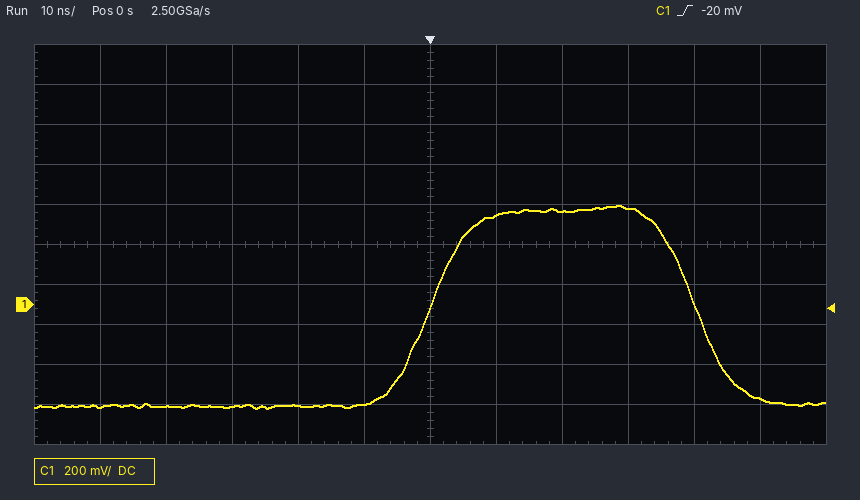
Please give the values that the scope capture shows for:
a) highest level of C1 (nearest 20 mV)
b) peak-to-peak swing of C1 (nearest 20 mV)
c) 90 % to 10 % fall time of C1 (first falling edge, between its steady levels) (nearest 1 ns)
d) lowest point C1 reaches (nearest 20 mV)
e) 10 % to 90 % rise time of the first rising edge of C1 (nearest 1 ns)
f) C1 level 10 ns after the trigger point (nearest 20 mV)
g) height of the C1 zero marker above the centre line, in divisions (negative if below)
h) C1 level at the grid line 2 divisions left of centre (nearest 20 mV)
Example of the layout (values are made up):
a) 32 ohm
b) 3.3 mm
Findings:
a) 500 mV
b) 1.02 V
c) 12 ns
d) -520 mV
e) 12 ns
f) 440 mV
g) -1.5 div
h) -500 mV
